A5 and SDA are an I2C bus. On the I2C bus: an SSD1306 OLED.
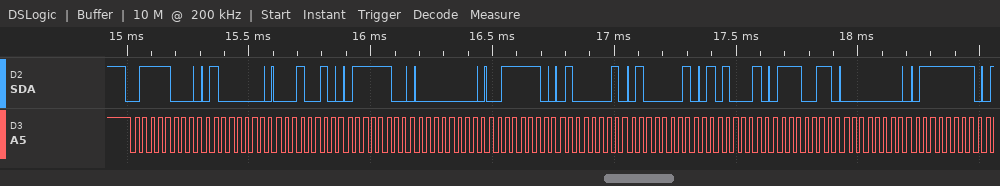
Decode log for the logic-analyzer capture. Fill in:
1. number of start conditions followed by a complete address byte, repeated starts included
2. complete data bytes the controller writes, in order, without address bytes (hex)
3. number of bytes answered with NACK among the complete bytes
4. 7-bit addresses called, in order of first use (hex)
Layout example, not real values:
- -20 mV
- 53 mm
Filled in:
- 1
- 40 12 7C 00 3E 41 41 51 73 00 7F
- 0
- 0x3C
